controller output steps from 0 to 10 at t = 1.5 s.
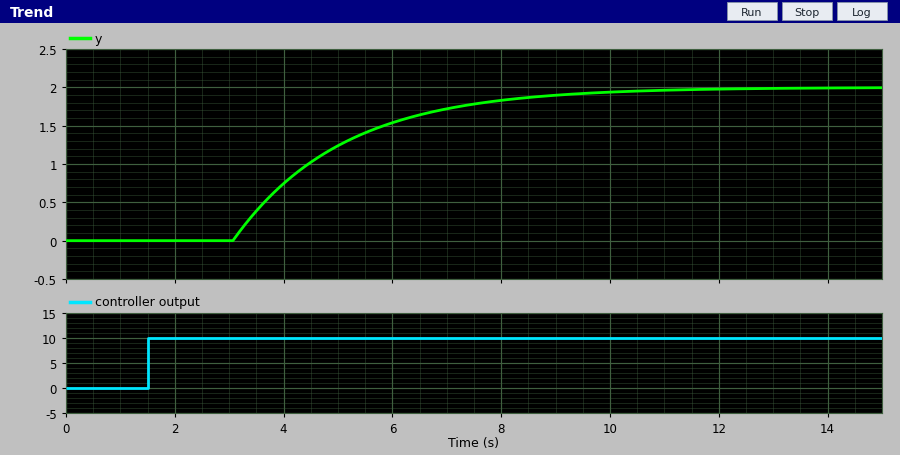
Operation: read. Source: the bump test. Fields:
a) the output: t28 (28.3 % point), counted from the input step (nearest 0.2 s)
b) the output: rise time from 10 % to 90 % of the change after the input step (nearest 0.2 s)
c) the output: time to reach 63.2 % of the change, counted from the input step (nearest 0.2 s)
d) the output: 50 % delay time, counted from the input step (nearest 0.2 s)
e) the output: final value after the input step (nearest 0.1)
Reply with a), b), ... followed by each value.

a) 2.2 s
b) 4.4 s
c) 3.6 s
d) 3.0 s
e) 2.0
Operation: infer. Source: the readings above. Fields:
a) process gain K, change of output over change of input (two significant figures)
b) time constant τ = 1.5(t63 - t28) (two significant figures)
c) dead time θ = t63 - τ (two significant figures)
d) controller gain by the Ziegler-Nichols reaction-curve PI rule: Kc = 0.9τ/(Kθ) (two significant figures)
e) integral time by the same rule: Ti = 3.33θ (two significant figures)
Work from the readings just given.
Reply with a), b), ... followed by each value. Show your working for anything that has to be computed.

a) (2 - 0) / 10 = 0.20
b) 1.5 × (3.6 - 2.2) = 2.1 s
c) 3.6 - 2.1 = 1.5 s
d) 0.9 × 2.1 / (0.2 × 1.5) = 6.3
e) 3.33 × 1.5 = 5.0 s
